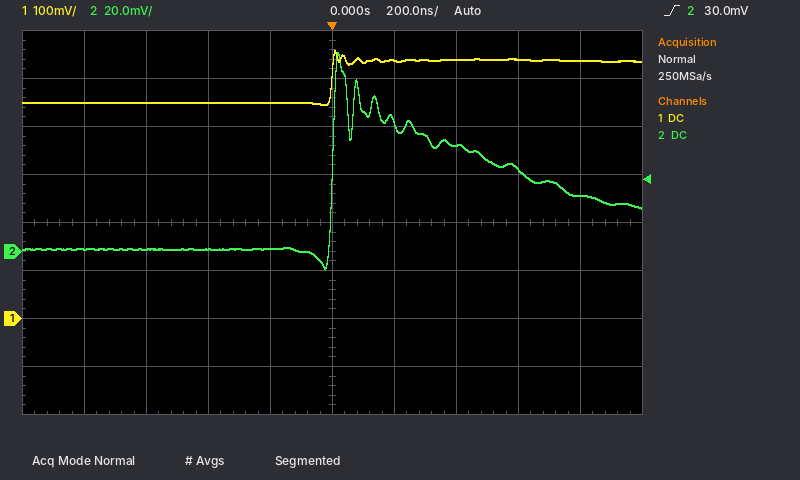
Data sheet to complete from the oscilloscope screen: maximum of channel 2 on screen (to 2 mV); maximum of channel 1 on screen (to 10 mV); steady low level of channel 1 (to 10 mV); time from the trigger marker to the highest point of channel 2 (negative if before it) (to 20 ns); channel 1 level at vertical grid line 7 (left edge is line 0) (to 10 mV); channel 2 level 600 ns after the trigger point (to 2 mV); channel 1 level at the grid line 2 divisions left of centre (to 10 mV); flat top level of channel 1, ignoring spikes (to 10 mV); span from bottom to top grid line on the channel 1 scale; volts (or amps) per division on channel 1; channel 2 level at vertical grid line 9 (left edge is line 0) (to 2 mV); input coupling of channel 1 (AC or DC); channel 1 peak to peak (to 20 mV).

82 mV
560 mV
450 mV
+20 ns
540 mV
34 mV
450 mV
540 mV
800 mV
100 mV
24 mV
DC
120 mV
